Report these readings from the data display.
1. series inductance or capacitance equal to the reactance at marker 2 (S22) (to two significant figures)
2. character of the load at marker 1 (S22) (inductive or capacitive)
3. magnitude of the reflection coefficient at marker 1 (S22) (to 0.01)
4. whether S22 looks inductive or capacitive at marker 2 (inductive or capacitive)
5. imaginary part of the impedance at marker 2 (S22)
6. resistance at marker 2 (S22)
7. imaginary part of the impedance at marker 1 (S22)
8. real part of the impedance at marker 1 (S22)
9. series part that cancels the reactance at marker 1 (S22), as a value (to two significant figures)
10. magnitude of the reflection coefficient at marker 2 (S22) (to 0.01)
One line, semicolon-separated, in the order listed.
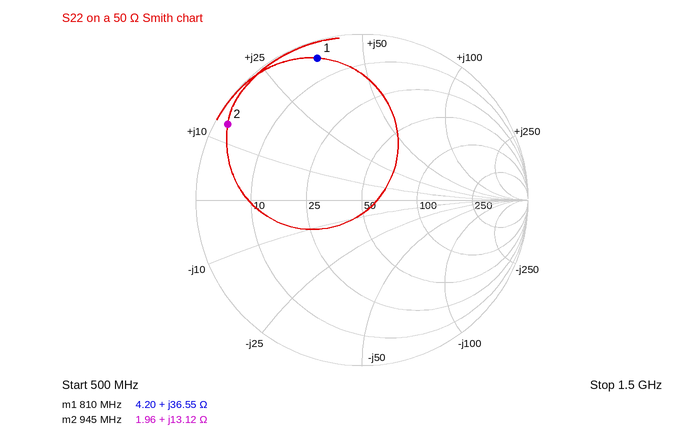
2.2 nH; inductive; 0.90; inductive; +13.12 Ω; 1.96 Ω; +36.55 Ω; 4.20 Ω; 5.4 pF; 0.93
